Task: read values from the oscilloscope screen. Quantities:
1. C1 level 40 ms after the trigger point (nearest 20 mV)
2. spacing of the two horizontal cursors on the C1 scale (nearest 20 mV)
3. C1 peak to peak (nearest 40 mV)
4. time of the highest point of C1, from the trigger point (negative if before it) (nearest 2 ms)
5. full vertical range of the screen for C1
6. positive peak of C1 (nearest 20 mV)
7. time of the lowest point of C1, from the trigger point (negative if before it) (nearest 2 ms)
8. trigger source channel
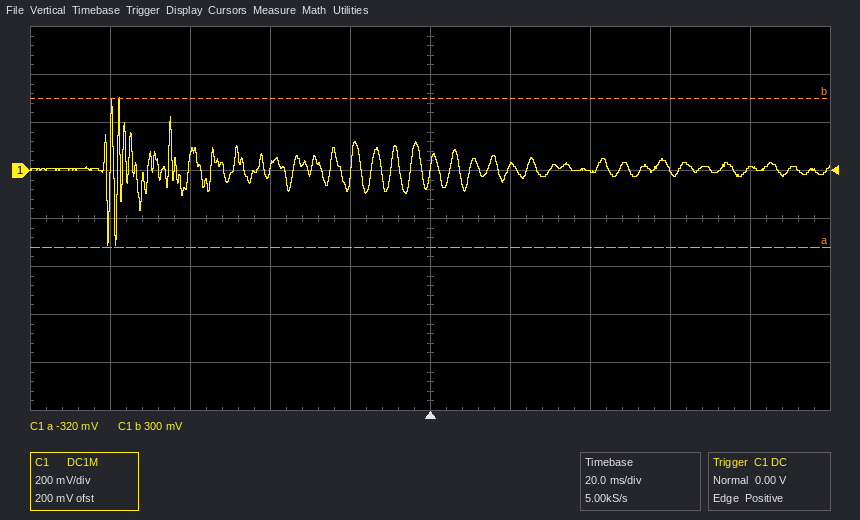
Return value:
0 mV
620 mV
600 mV
-78 ms
1.6 V
300 mV
-80 ms
C1
